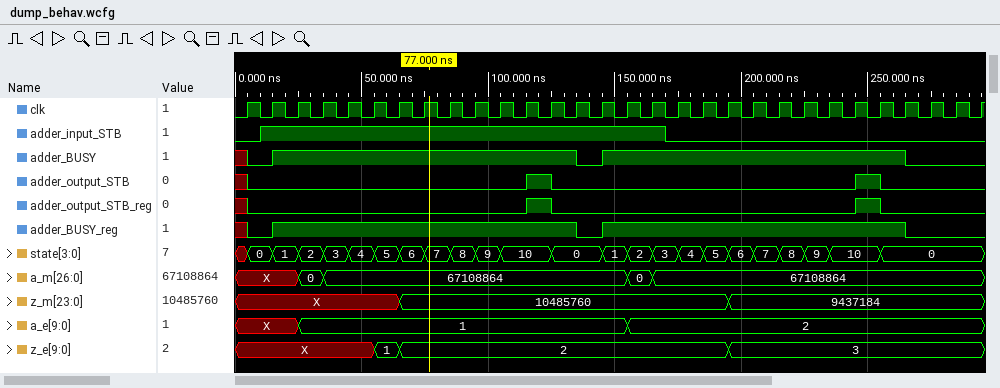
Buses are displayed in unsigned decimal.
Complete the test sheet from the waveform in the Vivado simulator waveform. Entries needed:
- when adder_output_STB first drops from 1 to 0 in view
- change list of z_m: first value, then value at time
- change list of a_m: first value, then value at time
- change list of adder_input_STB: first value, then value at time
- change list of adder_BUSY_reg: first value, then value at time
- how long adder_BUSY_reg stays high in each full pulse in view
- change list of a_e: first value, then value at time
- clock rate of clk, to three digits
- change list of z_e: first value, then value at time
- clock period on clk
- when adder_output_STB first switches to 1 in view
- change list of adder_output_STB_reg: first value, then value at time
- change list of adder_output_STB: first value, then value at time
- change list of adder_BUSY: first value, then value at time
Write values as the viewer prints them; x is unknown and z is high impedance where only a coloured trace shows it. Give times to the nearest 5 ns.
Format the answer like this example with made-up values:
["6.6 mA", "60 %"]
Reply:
["125 ns", "X, 10485760 at 65 ns, 9437184 at 195 ns", "X, 0 at 25 ns, 67108864 at 35 ns, 0 at 155 ns, 67108864 at 165 ns", "0, 1 at 10 ns, 0 at 170 ns", "x, 0 at 5 ns, 1 at 15 ns, 0 at 135 ns, 1 at 145 ns, 0 at 265 ns", "120 ns, 120 ns", "X, 1 at 25 ns, 2 at 155 ns", "100 MHz", "X, 1 at 55 ns, 2 at 65 ns, 3 at 195 ns", "10 ns", "115 ns", "x, 0 at 5 ns, 1 at 115 ns, 0 at 125 ns, 1 at 245 ns, 0 at 255 ns", "x, 0 at 5 ns, 1 at 115 ns, 0 at 125 ns, 1 at 245 ns, 0 at 255 ns", "x, 0 at 5 ns, 1 at 15 ns, 0 at 135 ns, 1 at 145 ns, 0 at 265 ns"]
